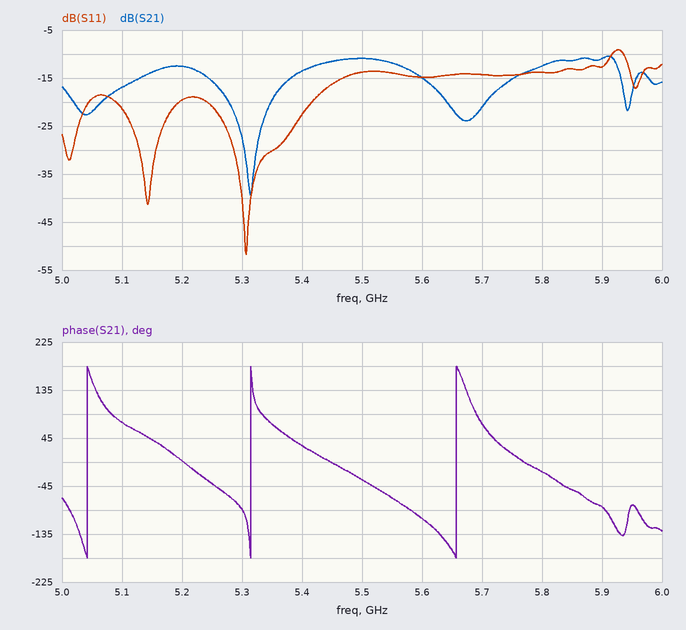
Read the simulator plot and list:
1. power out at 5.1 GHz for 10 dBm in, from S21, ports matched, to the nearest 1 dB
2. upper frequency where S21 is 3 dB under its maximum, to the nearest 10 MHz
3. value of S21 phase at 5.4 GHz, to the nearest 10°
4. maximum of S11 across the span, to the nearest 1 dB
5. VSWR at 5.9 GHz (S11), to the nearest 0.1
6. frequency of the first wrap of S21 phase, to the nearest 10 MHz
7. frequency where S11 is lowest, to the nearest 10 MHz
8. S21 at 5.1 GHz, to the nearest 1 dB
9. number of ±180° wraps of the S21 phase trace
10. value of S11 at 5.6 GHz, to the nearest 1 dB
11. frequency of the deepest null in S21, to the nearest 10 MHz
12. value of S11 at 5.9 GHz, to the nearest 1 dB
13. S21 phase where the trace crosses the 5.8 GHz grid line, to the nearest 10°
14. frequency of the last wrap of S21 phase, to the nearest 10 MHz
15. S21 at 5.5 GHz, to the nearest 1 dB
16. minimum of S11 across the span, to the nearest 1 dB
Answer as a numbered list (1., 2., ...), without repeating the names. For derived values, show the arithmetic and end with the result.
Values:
1. 10 dBm + (-17 dB) = -7 dBm
2. 5.93 GHz
3. 30°
4. -9 dB
5. |Γ| = 10^(-13/20) = 0.2239; VSWR = (1 + 0.2239)/(1 − 0.2239) ≈ 1.6
6. 5.04 GHz
7. 5.31 GHz
8. -17 dB
9. 3
10. -15 dB
11. 5.31 GHz
12. -13 dB
13. -20°
14. 5.66 GHz
15. -11 dB
16. -52 dB
